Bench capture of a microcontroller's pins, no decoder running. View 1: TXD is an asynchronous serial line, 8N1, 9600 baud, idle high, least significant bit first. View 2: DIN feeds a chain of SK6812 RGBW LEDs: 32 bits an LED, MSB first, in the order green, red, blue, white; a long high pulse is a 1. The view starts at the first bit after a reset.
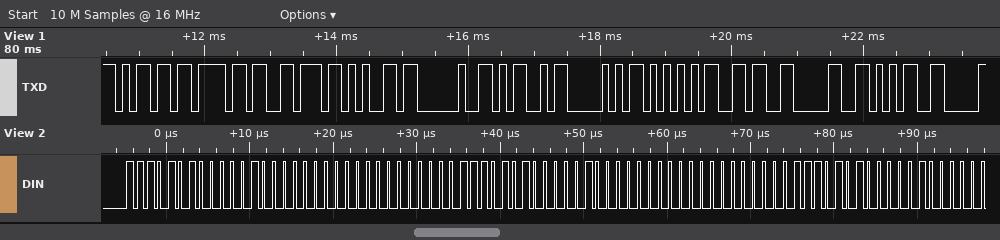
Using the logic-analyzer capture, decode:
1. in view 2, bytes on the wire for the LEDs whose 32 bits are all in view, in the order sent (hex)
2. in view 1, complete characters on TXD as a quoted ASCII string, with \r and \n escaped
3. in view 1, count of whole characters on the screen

EA 08 00 00 EA 08 00 00
"move MPU605"
11
